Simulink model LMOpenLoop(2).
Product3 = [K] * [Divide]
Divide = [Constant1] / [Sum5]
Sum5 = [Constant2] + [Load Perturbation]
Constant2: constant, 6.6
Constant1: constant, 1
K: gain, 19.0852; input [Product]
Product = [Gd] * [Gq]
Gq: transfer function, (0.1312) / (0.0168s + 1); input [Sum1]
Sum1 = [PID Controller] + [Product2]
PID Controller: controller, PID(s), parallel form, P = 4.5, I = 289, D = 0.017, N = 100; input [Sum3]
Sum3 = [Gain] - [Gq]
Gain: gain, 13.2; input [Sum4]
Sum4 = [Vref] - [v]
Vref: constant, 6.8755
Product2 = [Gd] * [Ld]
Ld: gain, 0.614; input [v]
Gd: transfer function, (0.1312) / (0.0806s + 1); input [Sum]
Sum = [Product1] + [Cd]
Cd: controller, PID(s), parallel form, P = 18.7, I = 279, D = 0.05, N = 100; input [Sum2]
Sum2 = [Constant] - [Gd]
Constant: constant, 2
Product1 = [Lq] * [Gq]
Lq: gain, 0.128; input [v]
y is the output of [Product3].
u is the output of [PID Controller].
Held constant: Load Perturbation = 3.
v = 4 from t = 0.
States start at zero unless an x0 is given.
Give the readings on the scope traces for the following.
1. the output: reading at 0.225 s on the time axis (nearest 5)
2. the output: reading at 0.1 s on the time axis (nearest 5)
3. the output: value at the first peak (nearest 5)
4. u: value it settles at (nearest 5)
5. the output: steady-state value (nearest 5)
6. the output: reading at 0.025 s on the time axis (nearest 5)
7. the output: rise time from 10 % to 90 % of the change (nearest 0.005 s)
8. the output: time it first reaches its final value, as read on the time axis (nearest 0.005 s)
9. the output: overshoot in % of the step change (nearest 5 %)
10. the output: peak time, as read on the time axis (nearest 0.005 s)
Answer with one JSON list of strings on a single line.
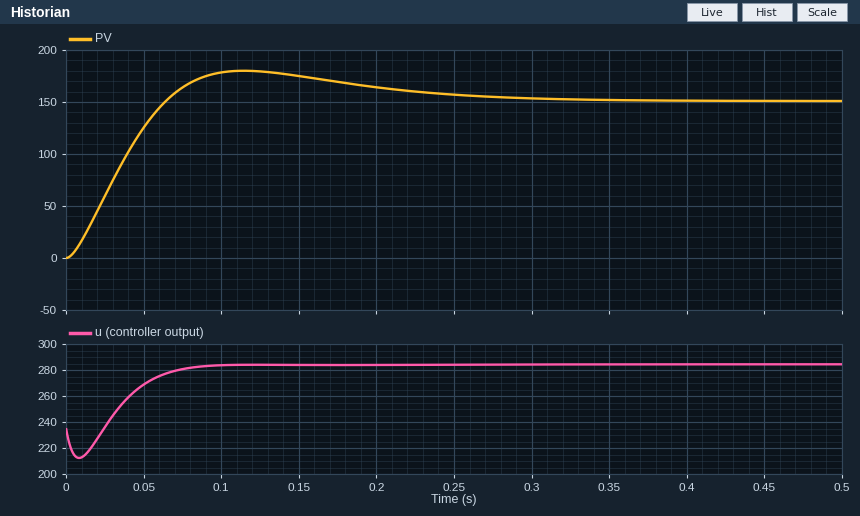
["160", "180", "180", "285", "150", "60", "0.045 s", "0.065 s", "20 %", "0.115 s"]
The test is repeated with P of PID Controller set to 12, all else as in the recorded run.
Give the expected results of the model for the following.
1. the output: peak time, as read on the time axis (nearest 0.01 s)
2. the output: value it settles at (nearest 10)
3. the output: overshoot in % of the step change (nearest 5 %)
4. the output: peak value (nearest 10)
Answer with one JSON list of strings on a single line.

["0.13 s", "150", "10 %", "170"]
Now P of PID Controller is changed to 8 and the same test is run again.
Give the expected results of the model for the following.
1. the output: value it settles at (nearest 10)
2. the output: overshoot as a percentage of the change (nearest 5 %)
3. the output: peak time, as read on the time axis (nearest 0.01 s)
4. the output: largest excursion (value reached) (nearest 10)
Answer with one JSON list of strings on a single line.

["150", "15 %", "0.12 s", "170"]
